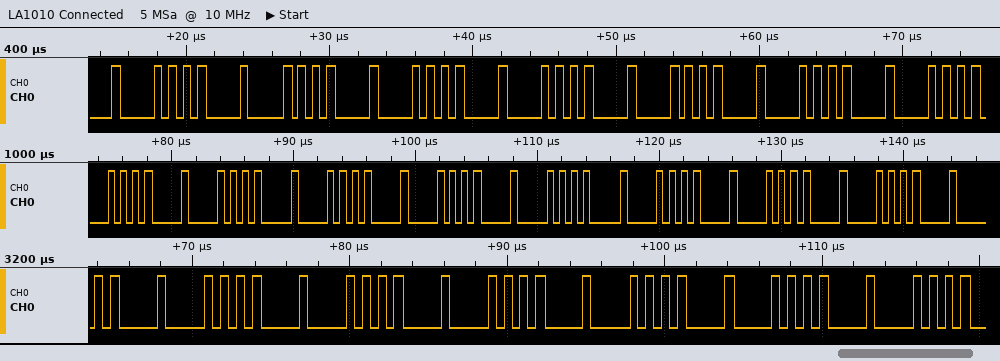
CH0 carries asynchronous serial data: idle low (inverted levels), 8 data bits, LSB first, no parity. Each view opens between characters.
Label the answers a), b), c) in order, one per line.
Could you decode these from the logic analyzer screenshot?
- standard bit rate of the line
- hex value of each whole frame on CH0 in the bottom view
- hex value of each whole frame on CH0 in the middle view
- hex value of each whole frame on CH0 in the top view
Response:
a) 2000000 baud
b) 7D, D5, 5F, 7D, D5, 5F, 7D, D5, 5F
c) D5, 5F, 7D, D5, 5F, 7D, D5, 5F, 7D, D5, 5F, 7D
d) 5F, 7D, D5, 5F, 7D, D5, 5F, 7D, D5, 5F
